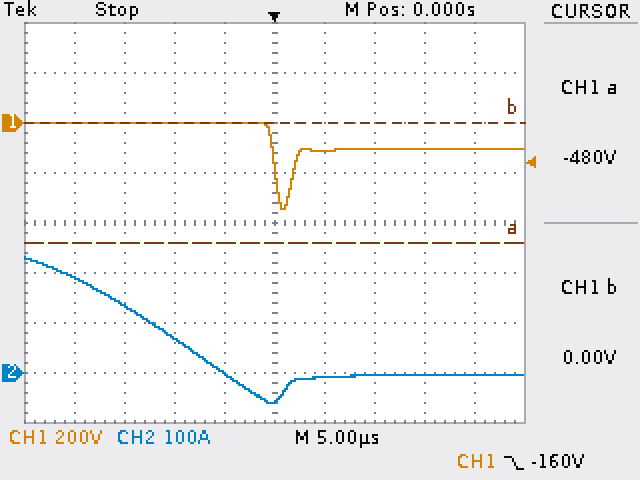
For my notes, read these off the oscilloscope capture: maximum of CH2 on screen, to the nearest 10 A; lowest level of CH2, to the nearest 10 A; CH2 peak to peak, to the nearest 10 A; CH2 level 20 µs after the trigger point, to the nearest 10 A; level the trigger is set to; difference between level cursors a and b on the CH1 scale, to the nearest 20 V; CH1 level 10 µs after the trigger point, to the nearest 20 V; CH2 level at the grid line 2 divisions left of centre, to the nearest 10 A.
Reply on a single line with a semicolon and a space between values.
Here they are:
230 A; -60 A; 290 A; 0 A; -160 V; 480 V; -100 V; 70 A
